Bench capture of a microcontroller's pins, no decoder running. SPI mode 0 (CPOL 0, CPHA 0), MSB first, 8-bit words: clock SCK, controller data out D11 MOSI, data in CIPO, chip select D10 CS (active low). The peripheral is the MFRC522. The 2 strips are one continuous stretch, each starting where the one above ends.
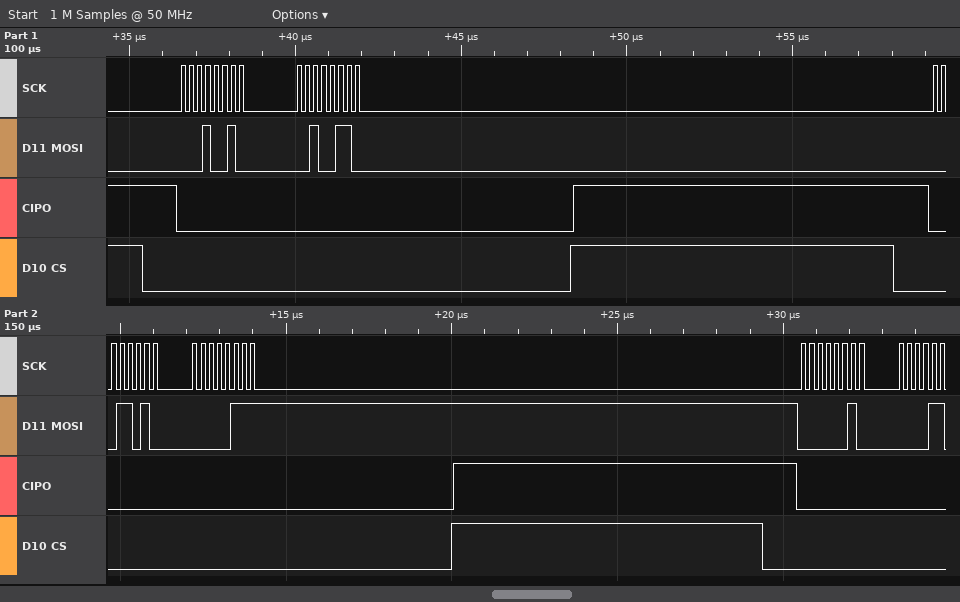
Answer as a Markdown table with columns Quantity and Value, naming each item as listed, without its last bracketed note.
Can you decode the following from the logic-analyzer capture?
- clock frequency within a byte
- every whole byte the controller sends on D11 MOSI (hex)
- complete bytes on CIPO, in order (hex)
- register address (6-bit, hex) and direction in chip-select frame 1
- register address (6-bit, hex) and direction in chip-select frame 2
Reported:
| Quantity | Value |
|---|---|
| clock frequency within a byte | 4 MHz |
| every whole byte the controller sends on D11 MOSI | 0x12 0x26 0x1A 0x07 0x02 |
| complete bytes on CIPO, in order | 0x00 0x00 0x00 0x00 0x00 |
| register address (6-bit, hex) and direction in chip-select frame 1 | 0x09 write |
| register address (6-bit, hex) and direction in chip-select frame 2 | 0x0D write |
